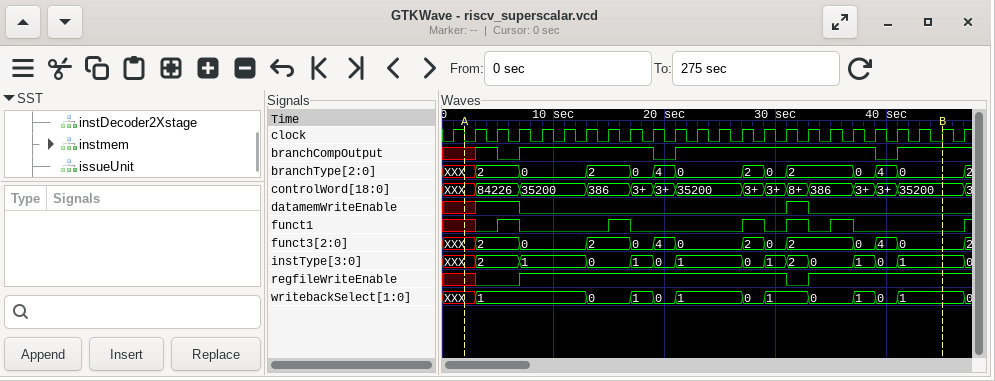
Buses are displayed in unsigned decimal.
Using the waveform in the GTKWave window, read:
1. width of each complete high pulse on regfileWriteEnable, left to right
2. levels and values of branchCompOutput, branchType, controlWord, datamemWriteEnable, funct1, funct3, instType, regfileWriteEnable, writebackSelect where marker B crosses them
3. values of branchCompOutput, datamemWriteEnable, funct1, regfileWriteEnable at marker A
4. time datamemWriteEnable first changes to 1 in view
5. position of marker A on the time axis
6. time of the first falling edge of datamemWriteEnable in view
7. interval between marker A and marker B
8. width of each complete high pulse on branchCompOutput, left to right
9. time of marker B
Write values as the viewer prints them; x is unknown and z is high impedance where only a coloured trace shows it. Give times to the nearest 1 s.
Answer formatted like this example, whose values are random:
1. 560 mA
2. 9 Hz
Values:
1. 24 s
2. branchCompOutput=1, branchType=0, controlWord=35200, datamemWriteEnable=0, funct1=0, funct3=0, instType=1, regfileWriteEnable=1, writebackSelect=1
3. branchCompOutput=x, datamemWriteEnable=x, funct1=x, regfileWriteEnable=x
4. 3 s
5. 2 s
6. 7 s
7. 43 s
8. 12 s, 18 s
9. 45 s
